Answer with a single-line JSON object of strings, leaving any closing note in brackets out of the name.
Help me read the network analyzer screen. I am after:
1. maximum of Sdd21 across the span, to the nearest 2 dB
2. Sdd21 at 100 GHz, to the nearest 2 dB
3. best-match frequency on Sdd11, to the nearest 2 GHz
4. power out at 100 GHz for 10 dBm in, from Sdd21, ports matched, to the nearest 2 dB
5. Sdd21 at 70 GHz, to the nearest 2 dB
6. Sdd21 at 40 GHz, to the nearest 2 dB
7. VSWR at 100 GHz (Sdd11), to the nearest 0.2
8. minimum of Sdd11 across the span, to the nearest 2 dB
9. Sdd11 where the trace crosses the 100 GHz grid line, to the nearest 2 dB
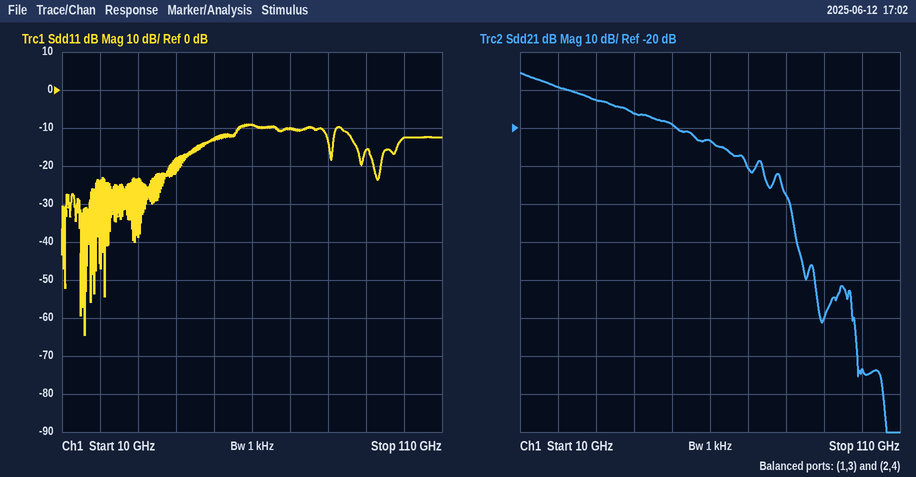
{"maximum of Sdd21 across the span, to the nearest 2 dB": "-6 dB", "Sdd21 at 100 GHz, to the nearest 2 dB": "-84 dB", "best-match frequency on Sdd11, to the nearest 2 GHz": "16 GHz", "power out at 100 GHz for 10 dBm in, from Sdd21, ports matched, to the nearest 2 dB": "-74 dBm", "Sdd21 at 70 GHz, to the nearest 2 dB": "-30 dB", "Sdd21 at 40 GHz, to the nearest 2 dB": "-16 dB", "VSWR at 100 GHz (Sdd11), to the nearest 0.2": "1.6", "minimum of Sdd11 across the span, to the nearest 2 dB": "-64 dB", "Sdd11 where the trace crosses the 100 GHz grid line, to the nearest 2 dB": "-12 dB"}
